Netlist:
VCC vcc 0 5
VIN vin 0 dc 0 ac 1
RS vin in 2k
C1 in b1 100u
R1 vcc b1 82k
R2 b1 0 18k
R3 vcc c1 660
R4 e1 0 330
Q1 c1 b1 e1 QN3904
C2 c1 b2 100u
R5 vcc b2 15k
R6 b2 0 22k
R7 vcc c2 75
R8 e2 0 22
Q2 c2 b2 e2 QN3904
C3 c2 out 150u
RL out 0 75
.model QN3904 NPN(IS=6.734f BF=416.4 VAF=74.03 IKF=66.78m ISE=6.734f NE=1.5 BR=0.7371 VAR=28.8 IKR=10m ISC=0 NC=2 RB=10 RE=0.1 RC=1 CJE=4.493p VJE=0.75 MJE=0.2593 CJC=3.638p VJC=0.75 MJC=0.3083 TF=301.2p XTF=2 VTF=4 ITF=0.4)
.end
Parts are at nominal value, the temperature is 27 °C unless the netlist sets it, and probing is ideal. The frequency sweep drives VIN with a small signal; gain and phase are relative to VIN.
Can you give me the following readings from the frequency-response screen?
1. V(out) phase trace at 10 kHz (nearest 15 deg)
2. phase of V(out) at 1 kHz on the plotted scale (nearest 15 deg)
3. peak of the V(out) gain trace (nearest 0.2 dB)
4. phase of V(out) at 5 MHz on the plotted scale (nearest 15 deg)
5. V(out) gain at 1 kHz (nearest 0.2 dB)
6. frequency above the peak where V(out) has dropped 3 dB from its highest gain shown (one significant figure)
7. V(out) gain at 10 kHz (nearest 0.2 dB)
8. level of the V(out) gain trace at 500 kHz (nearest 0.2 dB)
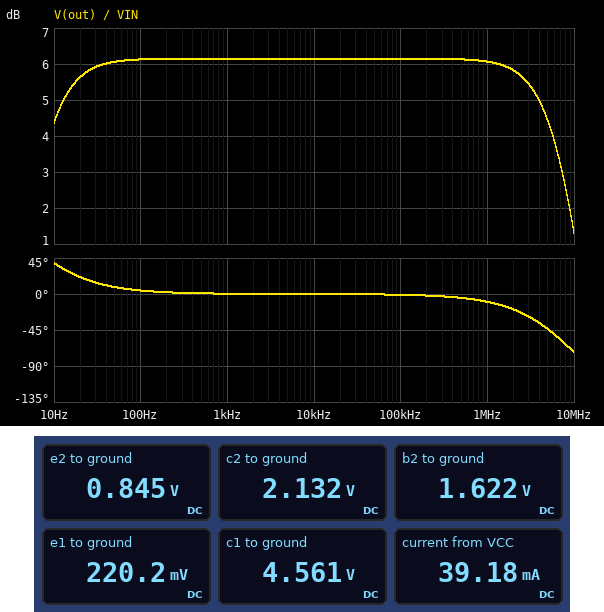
0 deg
0 deg
6.2 dB
-45 deg
6.2 dB
7 MHz
6.2 dB
6.2 dB
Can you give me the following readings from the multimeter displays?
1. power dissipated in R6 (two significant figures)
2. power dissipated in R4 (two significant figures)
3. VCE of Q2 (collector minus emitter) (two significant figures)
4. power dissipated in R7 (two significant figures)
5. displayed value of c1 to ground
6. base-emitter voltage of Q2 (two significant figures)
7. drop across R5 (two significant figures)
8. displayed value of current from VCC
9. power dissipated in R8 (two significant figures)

120 µW
150 µW
1.3 V
110 mW
4.561 V
780 mV
3.4 V
39.18 mA
32 mW
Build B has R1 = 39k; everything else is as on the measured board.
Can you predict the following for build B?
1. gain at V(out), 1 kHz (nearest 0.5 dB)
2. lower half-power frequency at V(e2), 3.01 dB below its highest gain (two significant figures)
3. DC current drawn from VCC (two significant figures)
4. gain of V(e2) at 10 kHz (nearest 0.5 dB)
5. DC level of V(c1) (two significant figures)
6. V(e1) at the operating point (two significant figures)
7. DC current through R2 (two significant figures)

6.5 dB
490 mHz
41 mA
2.0 dB
3.4 V
810 mV
83 µA
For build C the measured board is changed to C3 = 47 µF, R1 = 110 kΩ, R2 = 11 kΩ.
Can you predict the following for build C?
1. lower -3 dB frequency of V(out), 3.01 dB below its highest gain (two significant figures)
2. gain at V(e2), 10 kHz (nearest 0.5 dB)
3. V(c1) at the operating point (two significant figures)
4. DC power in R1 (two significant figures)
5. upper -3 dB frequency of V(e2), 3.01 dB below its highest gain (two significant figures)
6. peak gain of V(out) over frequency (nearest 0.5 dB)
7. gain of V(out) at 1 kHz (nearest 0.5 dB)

4.6 MHz
-46.0 dB
5.0 V
190 µW
29 MHz
-25.5 dB
-41.5 dB
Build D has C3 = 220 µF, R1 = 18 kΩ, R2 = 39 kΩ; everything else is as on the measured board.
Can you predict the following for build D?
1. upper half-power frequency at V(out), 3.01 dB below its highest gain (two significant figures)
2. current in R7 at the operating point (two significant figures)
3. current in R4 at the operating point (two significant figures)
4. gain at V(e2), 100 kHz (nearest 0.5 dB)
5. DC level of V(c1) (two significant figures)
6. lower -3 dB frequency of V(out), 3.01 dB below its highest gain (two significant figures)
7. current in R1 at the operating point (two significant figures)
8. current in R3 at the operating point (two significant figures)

120 MHz
38 mA
5.0 mA
-49.5 dB
1.8 V
18 MHz
150 µA
4.9 mA
